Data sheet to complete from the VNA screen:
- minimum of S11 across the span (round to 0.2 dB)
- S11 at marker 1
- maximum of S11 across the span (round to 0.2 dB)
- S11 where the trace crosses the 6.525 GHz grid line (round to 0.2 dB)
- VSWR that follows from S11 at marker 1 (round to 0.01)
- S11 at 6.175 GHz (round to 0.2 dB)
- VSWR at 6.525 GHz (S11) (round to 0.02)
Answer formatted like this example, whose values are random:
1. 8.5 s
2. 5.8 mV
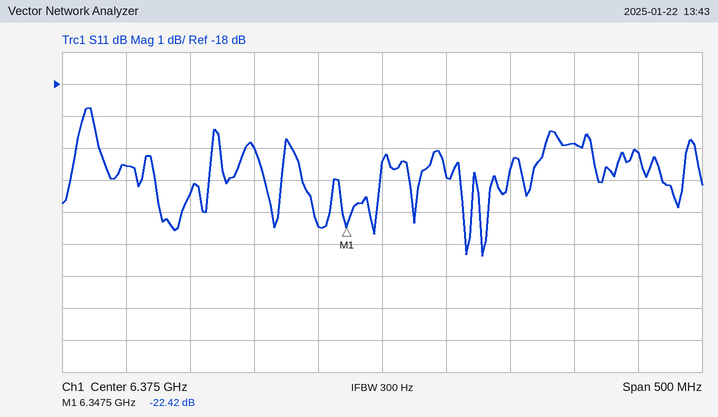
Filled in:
1. -23.4 dB
2. -22.42 dB
3. -18.8 dB
4. -19.8 dB
5. 1.16
6. -20.6 dB
7. 1.22
